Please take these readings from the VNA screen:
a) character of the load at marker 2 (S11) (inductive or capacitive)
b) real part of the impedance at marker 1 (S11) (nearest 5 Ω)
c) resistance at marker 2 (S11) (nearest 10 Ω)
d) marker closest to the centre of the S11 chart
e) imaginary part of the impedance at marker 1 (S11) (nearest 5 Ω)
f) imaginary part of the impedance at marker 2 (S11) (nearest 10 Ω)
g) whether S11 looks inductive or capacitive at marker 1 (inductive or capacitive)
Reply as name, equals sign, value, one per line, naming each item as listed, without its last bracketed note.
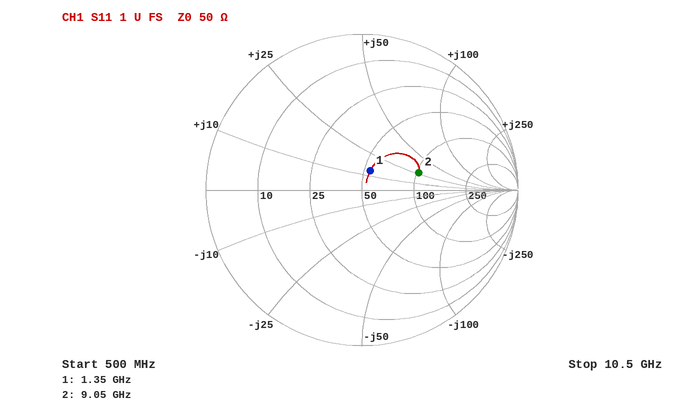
character of the load at marker 2 (S11) = inductive
real part of the impedance at marker 1 (S11) = 55 Ω
resistance at marker 2 (S11) = 100 Ω
marker closest to the centre of the S11 chart = marker 1
imaginary part of the impedance at marker 1 (S11) = +15 Ω
imaginary part of the impedance at marker 2 (S11) = +30 Ω
whether S11 looks inductive or capacitive at marker 1 = inductive
